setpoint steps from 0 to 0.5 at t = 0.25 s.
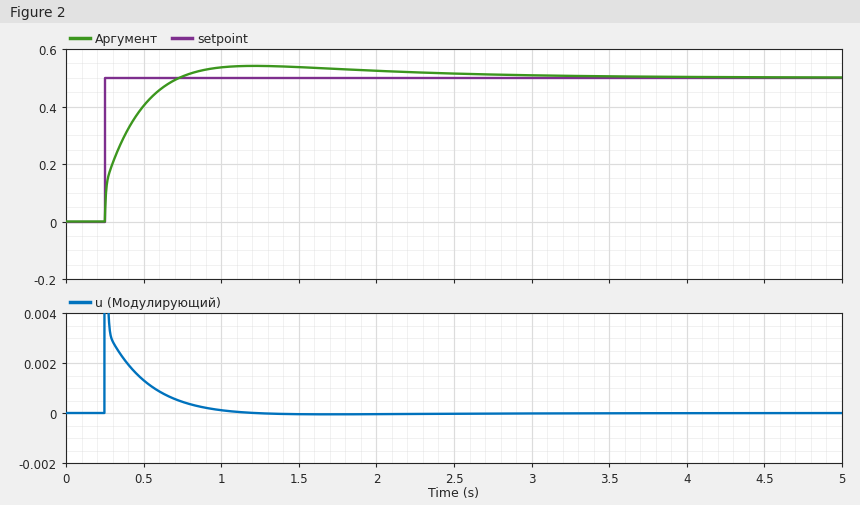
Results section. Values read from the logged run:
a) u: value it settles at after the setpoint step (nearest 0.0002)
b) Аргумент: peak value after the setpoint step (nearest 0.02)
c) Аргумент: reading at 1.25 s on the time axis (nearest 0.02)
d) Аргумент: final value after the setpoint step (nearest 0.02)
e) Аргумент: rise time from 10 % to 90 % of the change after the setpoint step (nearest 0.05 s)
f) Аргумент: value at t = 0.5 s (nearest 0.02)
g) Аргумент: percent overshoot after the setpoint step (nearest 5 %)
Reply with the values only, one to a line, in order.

0.0000
0.54
0.54
0.50
0.35 s
0.40
10 %
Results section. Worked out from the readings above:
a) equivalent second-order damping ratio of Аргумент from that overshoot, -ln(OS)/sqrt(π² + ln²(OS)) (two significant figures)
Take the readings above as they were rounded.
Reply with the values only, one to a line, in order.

0.59
